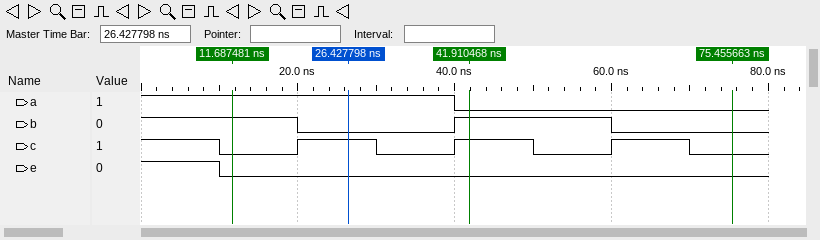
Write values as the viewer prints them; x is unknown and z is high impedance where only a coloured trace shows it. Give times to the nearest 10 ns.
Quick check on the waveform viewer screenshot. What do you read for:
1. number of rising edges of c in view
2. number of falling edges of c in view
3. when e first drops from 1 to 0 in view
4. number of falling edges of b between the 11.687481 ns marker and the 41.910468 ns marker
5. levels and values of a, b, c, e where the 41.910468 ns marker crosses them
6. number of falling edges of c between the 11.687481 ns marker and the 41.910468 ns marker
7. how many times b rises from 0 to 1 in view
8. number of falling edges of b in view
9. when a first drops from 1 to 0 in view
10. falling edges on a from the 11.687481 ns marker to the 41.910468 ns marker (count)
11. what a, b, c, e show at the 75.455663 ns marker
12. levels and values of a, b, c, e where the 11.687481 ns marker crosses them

3
4
10 ns
1
a=0, b=1, c=1, e=0
1
1
2
40 ns
1
a=0, b=0, c=0, e=0
a=1, b=1, c=0, e=0
